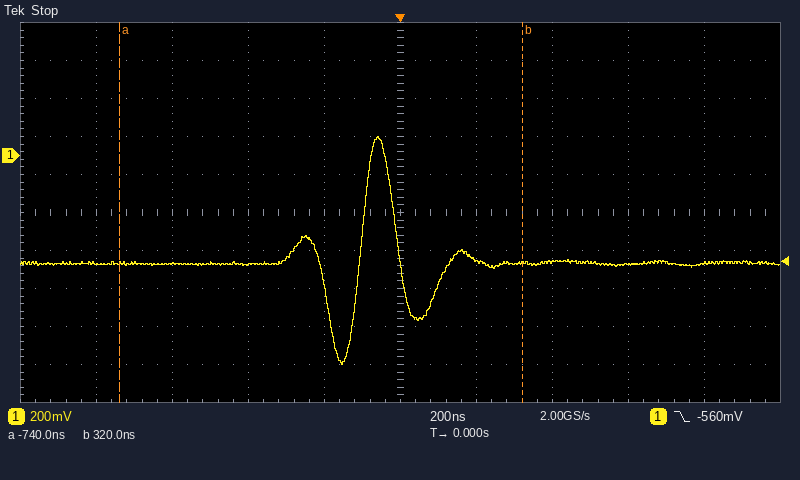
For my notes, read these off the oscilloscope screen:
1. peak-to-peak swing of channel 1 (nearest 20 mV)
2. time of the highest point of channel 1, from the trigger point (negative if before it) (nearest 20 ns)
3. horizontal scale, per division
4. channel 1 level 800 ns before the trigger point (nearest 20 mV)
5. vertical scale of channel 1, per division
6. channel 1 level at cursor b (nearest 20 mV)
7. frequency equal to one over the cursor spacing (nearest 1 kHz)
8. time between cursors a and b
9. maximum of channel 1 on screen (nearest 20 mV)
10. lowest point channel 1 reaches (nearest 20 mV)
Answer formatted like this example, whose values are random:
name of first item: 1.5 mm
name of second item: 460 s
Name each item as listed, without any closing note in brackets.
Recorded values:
peak-to-peak swing of channel 1: 1.20 V
time of the highest point of channel 1, from the trigger point (negative if before it): -60 ns
horizontal scale, per division: 200 ns
channel 1 level 800 ns before the trigger point: -560 mV
vertical scale of channel 1, per division: 200 mV
channel 1 level at cursor b: -560 mV
frequency equal to one over the cursor spacing: 943 kHz
time between cursors a and b: 1.06 µs
maximum of channel 1 on screen: 100 mV
lowest point channel 1 reaches: -1.10 V
